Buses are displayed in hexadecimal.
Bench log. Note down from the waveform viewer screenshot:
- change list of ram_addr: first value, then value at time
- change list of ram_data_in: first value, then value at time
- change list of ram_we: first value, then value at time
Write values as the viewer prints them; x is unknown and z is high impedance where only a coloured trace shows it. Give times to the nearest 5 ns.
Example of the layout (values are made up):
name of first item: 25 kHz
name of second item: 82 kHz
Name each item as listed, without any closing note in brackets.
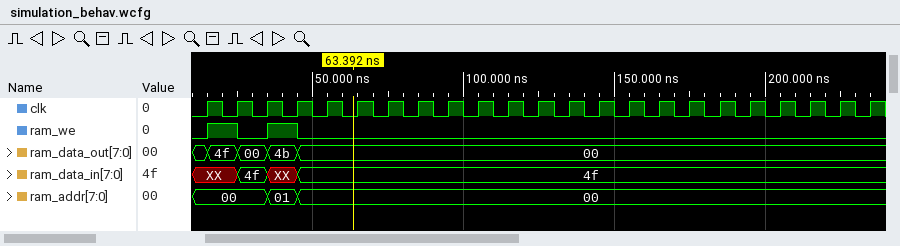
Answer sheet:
change list of ram_addr: first value, then value at time: 00, 01 at 35 ns, 00 at 45 ns
change list of ram_data_in: first value, then value at time: XX, 4f at 25 ns, XX at 35 ns, 4f at 45 ns
change list of ram_we: first value, then value at time: 0, 1 at 15 ns, 0 at 25 ns, 1 at 35 ns, 0 at 45 ns
